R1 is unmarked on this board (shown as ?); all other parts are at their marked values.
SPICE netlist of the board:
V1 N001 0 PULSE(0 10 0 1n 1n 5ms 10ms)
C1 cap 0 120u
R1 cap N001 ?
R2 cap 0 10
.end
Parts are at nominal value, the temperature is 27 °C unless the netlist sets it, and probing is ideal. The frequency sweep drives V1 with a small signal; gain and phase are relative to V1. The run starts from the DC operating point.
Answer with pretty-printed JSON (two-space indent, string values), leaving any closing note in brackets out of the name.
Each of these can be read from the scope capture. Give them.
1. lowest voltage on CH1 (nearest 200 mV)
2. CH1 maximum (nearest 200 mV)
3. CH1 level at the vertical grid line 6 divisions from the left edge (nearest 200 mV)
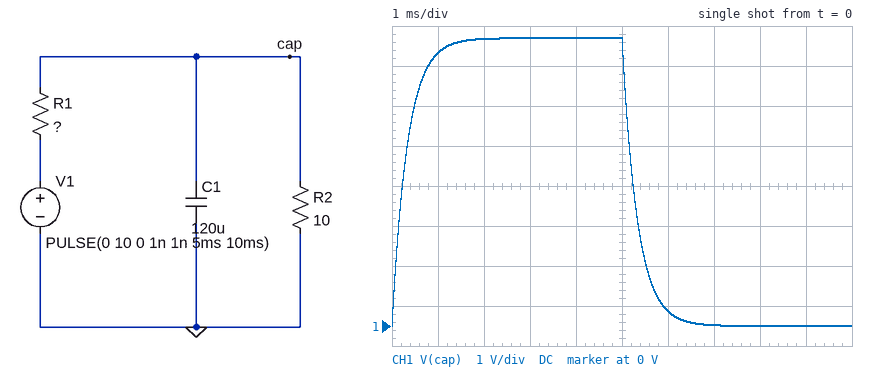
{
  "lowest voltage on CH1": "0 V",
  "CH1 maximum": "7.2 V",
  "CH1 level at the vertical grid line 6 divisions from the left edge": "400 mV"
}
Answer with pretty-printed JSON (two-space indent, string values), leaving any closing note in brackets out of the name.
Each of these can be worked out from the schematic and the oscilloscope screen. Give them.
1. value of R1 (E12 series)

{
  "value of R1": "3.9 Ω"
}
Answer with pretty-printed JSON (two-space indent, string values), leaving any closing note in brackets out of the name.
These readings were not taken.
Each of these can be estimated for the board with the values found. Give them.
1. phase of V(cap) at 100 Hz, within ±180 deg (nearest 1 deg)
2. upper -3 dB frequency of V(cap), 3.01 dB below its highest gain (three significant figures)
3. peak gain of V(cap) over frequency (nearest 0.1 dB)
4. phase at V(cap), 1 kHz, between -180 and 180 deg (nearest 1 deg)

{
  "phase of V(cap) at 100 Hz, within ±180 deg": "-12 deg",
  "upper -3 dB frequency of V(cap), 3.01 dB below its highest gain": "473 Hz",
  "peak gain of V(cap) over frequency": "-2.9 dB",
  "phase at V(cap), 1 kHz, between -180 and 180 deg": "-65 deg"
}
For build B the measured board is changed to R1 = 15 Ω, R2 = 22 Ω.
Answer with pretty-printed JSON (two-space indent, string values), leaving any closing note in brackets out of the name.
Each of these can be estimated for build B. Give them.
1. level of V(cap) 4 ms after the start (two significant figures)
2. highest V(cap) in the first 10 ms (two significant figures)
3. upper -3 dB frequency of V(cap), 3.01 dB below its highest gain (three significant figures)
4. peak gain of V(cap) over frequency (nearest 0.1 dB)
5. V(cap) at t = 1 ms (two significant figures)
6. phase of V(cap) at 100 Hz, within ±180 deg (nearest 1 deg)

{
  "level of V(cap) 4 ms after the start": "5.8 V",
  "highest V(cap) in the first 10 ms": "5.9 V",
  "upper -3 dB frequency of V(cap), 3.01 dB below its highest gain": "149 Hz",
  "peak gain of V(cap) over frequency": "-4.5 dB",
  "V(cap) at t = 1 ms": "3.6 V",
  "phase of V(cap) at 100 Hz, within ±180 deg": "-34 deg"
}
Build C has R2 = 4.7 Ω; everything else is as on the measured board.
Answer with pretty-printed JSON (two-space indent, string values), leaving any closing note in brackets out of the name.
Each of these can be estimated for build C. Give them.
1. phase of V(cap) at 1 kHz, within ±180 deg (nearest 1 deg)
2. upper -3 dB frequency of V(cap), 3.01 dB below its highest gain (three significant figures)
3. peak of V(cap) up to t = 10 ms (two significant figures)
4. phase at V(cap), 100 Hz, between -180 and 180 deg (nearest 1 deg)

{
  "phase of V(cap) at 1 kHz, within ±180 deg": "-58 deg",
  "upper -3 dB frequency of V(cap), 3.01 dB below its highest gain": "622 Hz",
  "peak of V(cap) up to t = 10 ms": "5.5 V",
  "phase at V(cap), 100 Hz, between -180 and 180 deg": "-9 deg"
}
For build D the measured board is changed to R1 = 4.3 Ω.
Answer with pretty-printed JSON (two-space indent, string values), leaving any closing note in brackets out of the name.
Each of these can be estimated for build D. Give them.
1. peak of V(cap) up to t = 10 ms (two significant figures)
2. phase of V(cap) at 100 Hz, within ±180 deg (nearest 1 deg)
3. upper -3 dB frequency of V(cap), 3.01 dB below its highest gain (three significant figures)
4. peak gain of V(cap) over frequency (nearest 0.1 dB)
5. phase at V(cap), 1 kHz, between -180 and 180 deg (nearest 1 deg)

{
  "peak of V(cap) up to t = 10 ms": "7.0 V",
  "phase of V(cap) at 100 Hz, within ±180 deg": "-13 deg",
  "upper -3 dB frequency of V(cap), 3.01 dB below its highest gain": "441 Hz",
  "peak gain of V(cap) over frequency": "-3.1 dB",
  "phase at V(cap), 1 kHz, between -180 and 180 deg": "-66 deg"
}
